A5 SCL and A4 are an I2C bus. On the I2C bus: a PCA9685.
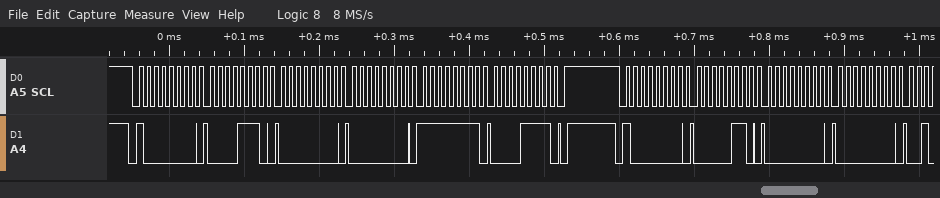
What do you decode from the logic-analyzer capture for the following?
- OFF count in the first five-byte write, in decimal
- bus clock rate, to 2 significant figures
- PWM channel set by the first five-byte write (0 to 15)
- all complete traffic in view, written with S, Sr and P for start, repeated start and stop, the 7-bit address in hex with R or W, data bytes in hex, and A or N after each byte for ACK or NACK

4095
100 kHz
2
S 40W A 0E A 00 A 00 A FF A 0F A P S 40W A 06 A 00 A 00 A
